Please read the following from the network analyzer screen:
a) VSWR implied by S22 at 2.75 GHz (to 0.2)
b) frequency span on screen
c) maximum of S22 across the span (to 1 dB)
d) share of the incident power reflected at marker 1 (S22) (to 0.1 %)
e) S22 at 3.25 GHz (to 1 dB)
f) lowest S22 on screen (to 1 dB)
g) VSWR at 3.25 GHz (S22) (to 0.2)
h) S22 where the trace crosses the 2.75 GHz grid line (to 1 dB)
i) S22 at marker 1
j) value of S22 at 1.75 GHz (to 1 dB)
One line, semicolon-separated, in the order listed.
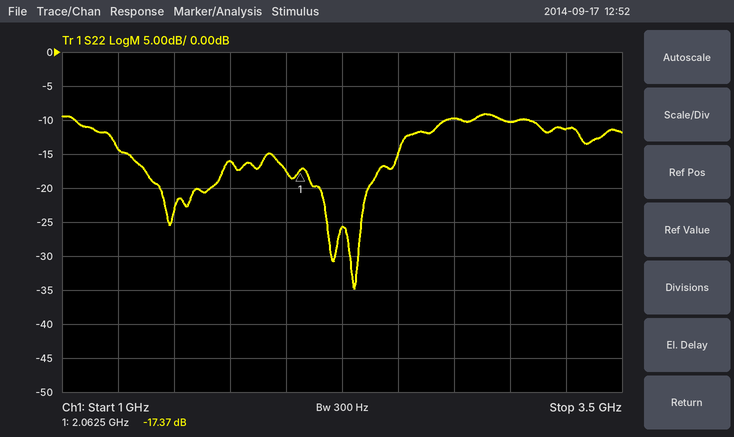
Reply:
2.0; 2.5 GHz; -9 dB; 1.8 %; -11 dB; -35 dB; 1.8; -10 dB; -17.37 dB; -16 dB
